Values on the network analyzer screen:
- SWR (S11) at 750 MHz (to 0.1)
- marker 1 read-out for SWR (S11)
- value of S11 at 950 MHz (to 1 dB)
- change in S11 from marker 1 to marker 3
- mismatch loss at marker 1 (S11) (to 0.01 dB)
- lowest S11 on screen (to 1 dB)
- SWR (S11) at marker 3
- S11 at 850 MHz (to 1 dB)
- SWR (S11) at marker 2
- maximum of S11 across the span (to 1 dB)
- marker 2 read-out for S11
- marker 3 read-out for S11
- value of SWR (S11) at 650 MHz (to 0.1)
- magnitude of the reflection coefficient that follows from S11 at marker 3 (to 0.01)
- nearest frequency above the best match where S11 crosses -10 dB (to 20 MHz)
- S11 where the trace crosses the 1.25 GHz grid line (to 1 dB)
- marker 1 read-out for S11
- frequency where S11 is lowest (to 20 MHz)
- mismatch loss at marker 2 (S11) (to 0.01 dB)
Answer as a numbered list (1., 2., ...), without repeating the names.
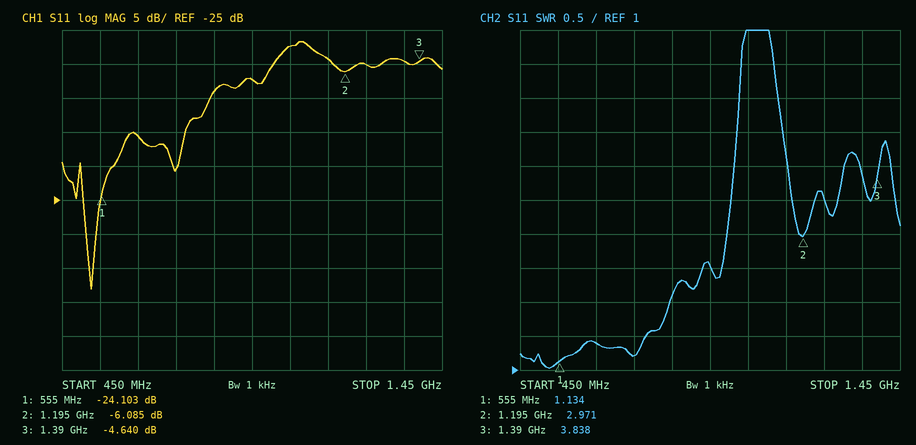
1. 1.2
2. 1.134
3. -7 dB
4. 19.463 dB
5. 0.02 dB
6. -38 dB
7. 3.838
8. -9 dB
9. 2.971
10. -2 dB
11. -6.085 dB
12. -4.640 dB
13. 1.4
14. 0.59
15. 840 MHz
16. -5 dB
17. -24.103 dB
18. 520 MHz
19. 1.23 dB
